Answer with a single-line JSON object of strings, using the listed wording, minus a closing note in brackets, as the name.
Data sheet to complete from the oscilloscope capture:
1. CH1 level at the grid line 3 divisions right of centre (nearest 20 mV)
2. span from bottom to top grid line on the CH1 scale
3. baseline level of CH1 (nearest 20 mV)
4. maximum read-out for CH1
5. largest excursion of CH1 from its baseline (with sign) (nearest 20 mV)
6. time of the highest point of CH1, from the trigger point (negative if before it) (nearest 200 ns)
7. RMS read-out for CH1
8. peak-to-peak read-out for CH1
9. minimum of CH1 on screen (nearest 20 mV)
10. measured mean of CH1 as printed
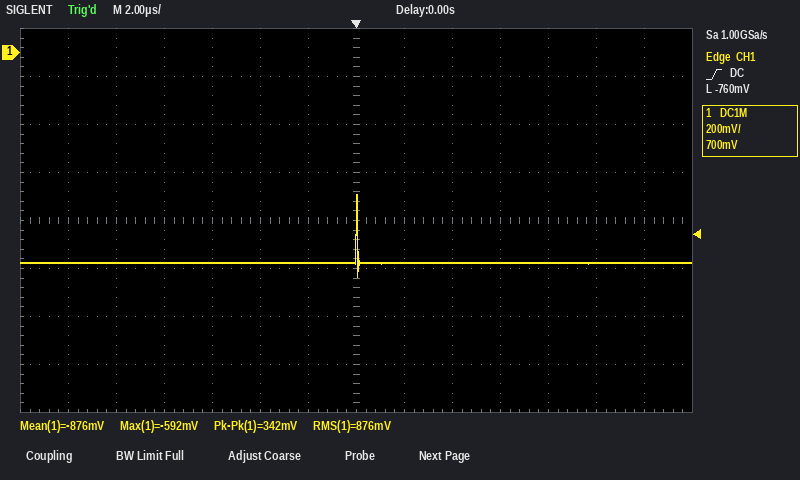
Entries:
{"CH1 level at the grid line 3 divisions right of centre": "-880 mV", "span from bottom to top grid line on the CH1 scale": "1.6 V", "baseline level of CH1": "-880 mV", "maximum read-out for CH1": "-592 mV", "largest excursion of CH1 from its baseline (with sign)": "+280 mV", "time of the highest point of CH1, from the trigger point (negative if before it)": "0.0 µs", "RMS read-out for CH1": "876 mV", "peak-to-peak read-out for CH1": "342 mV", "minimum of CH1 on screen": "-940 mV", "measured mean of CH1 as printed": "-876 mV"}
